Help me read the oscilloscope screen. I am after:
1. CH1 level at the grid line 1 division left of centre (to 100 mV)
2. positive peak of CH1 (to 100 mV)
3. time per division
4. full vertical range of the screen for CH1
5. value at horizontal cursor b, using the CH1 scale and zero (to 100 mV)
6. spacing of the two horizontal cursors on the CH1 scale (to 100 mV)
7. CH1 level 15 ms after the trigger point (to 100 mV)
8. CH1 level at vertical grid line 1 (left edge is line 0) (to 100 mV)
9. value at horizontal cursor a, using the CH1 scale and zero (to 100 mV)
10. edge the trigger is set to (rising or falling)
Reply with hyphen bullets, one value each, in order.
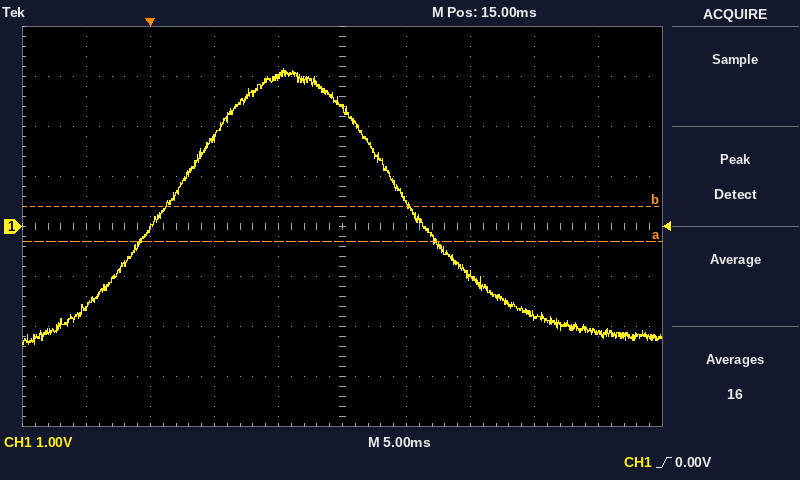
- 3.0 V
- 3.2 V
- 5 ms
- 8 V
- 400 mV
- 700 mV
- 2.3 V
- -1.6 V
- -300 mV
- rising
